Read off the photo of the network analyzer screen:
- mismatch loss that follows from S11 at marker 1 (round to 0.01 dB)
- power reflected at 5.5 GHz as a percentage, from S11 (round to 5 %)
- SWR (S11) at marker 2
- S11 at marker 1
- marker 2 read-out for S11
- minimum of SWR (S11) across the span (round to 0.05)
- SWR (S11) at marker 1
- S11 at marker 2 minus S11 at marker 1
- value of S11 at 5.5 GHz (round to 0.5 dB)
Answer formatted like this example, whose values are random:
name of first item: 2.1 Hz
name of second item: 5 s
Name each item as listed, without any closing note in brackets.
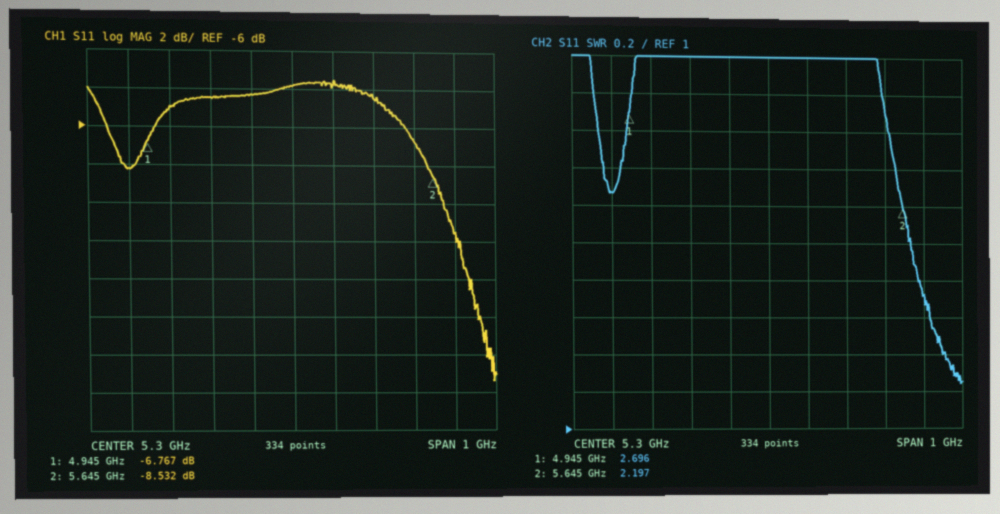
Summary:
mismatch loss that follows from S11 at marker 1: 1.03 dB
power reflected at 5.5 GHz as a percentage, from S11: 35 %
SWR (S11) at marker 2: 2.197
S11 at marker 1: -6.767 dB
marker 2 read-out for S11: -8.532 dB
minimum of SWR (S11) across the span: 1.25
SWR (S11) at marker 1: 2.696
S11 at marker 2 minus S11 at marker 1: -1.765 dB
value of S11 at 5.5 GHz: -4.5 dB
